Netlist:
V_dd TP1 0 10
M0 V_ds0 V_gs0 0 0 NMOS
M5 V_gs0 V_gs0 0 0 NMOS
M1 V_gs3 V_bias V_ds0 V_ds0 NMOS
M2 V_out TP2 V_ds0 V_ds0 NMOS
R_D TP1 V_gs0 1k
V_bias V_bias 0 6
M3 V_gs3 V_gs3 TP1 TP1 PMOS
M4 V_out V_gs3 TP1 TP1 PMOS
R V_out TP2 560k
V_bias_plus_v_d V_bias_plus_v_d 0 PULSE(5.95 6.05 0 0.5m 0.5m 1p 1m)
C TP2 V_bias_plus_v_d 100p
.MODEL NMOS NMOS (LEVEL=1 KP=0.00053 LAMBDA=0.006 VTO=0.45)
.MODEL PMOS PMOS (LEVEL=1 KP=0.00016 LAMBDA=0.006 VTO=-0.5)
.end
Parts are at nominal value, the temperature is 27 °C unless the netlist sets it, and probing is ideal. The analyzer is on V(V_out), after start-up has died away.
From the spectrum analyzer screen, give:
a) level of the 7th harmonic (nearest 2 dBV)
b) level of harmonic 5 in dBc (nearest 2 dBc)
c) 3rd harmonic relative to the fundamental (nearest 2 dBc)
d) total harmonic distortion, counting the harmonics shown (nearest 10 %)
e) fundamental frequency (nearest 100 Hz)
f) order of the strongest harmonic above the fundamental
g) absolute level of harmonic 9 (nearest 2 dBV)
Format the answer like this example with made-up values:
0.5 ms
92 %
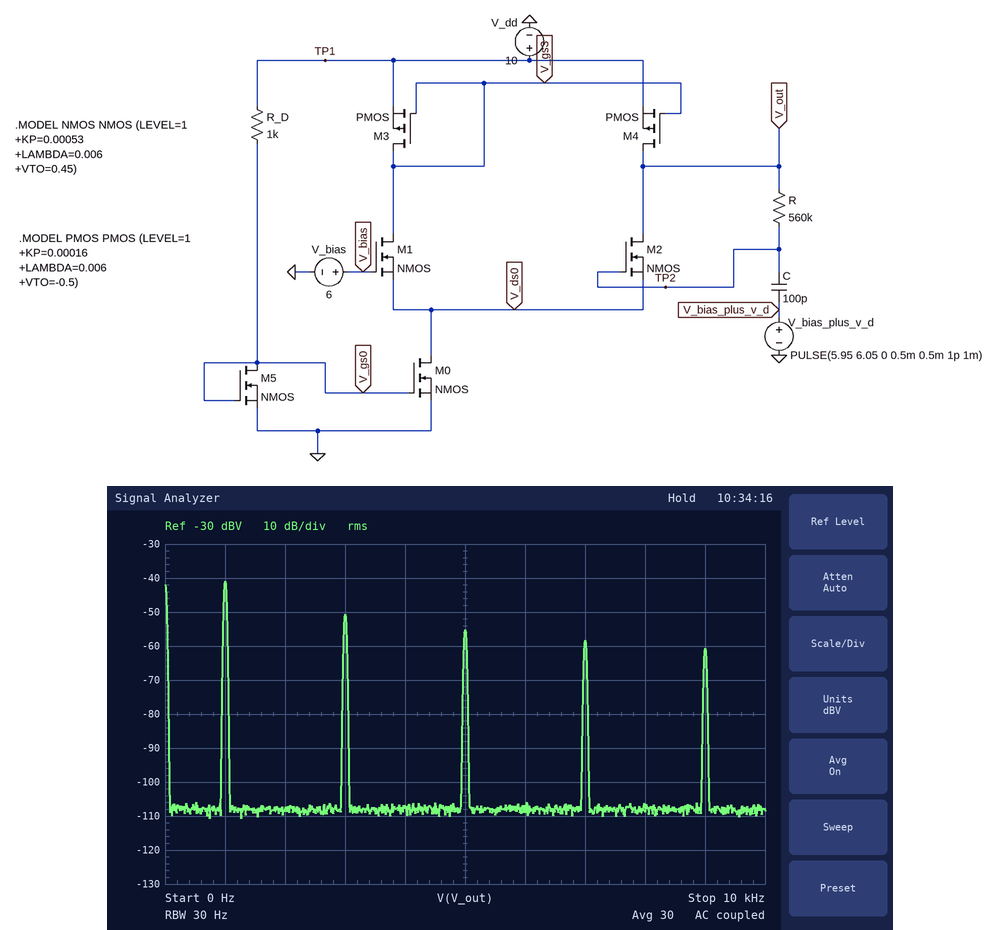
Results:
-58 dBV
-14 dBc
-10 dBc
40 %
1.0 kHz
3
-60 dBV
